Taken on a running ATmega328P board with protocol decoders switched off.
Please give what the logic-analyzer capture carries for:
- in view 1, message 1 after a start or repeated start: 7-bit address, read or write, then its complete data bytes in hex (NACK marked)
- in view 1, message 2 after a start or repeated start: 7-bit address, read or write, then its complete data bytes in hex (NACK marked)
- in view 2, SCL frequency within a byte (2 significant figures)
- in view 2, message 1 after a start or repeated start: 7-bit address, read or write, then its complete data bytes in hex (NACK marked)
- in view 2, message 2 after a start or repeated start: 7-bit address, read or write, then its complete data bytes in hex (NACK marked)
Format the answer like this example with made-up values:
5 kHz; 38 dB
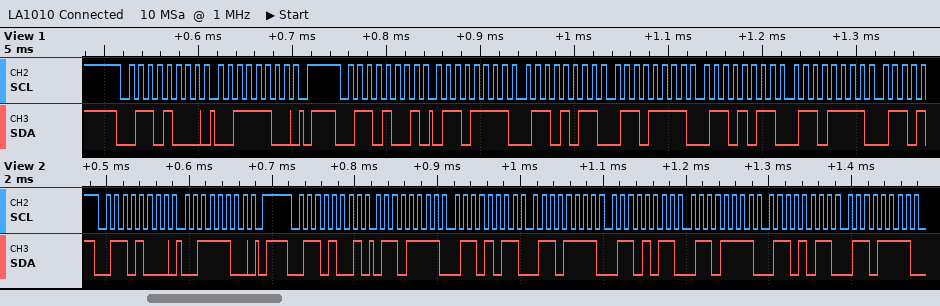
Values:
0x34 write: 3C; 0x34 read: 6F 6B 6F 6B 6F; 100 kHz; 0x34 write: 3C; 0x34 read: 6F 6B 6F 6B 6F 6B 6F
